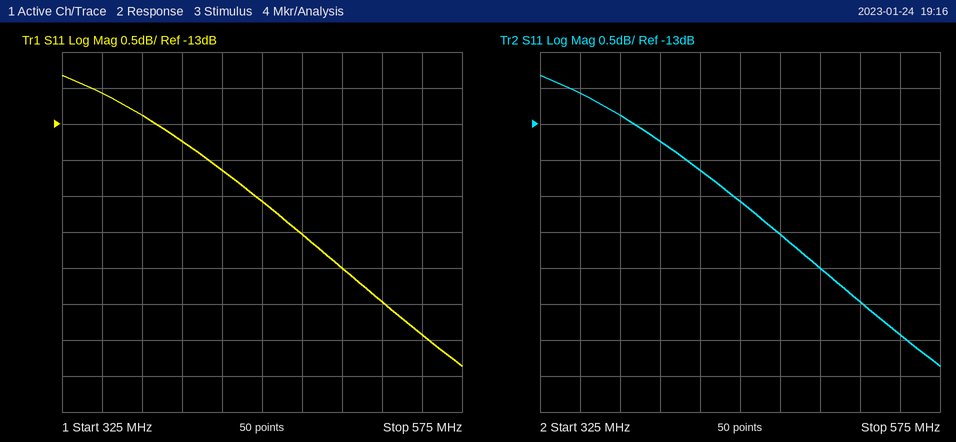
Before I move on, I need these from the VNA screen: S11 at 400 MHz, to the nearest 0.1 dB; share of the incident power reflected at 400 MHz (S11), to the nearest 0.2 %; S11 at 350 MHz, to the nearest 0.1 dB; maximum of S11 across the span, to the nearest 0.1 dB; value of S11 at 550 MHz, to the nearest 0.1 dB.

-13.2 dB
4.8 %
-12.6 dB
-12.3 dB
-15.9 dB
